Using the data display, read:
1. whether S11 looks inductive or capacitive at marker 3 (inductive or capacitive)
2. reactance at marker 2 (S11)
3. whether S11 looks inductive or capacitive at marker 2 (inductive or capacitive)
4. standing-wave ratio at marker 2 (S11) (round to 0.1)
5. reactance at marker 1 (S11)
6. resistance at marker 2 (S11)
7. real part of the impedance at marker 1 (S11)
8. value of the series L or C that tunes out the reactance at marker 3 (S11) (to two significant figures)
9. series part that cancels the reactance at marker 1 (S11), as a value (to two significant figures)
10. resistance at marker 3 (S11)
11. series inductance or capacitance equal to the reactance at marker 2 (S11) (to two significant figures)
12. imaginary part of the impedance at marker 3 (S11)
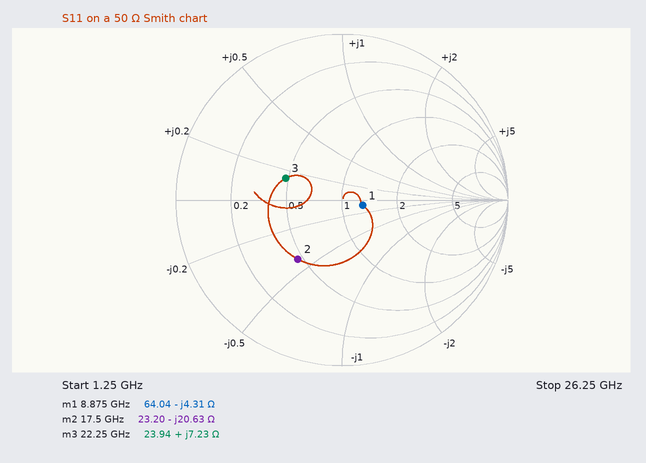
inductive
-20.63 Ω
capacitive
2.6
-4.31 Ω
23.20 Ω
64.04 Ω
990 fF
77 pH
23.94 Ω
440 fF
+7.23 Ω
